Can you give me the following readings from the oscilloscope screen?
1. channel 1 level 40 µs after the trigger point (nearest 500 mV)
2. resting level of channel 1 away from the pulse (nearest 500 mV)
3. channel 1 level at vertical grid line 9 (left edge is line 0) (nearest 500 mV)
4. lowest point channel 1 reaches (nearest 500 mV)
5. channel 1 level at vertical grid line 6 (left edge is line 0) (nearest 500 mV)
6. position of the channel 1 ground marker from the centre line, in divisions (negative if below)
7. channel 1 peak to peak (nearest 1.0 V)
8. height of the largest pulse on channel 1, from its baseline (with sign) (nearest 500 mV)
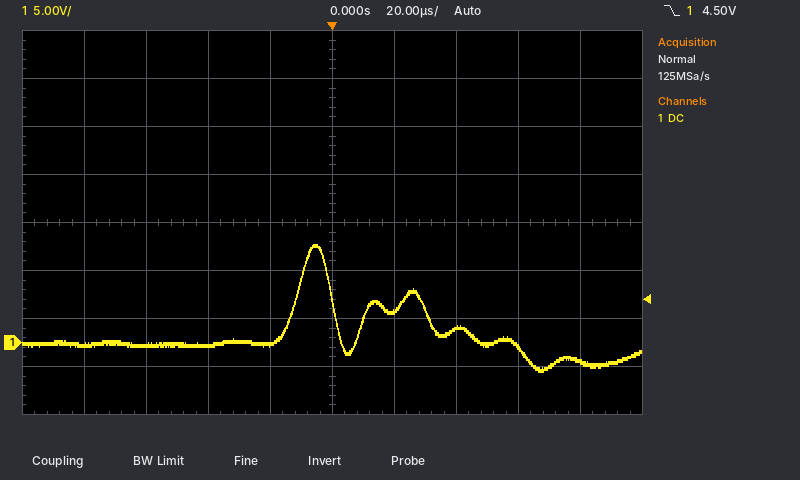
1.5 V
0.0 V
-2.0 V
-3.0 V
3.5 V
-2.5 div
13.0 V
+10.5 V
